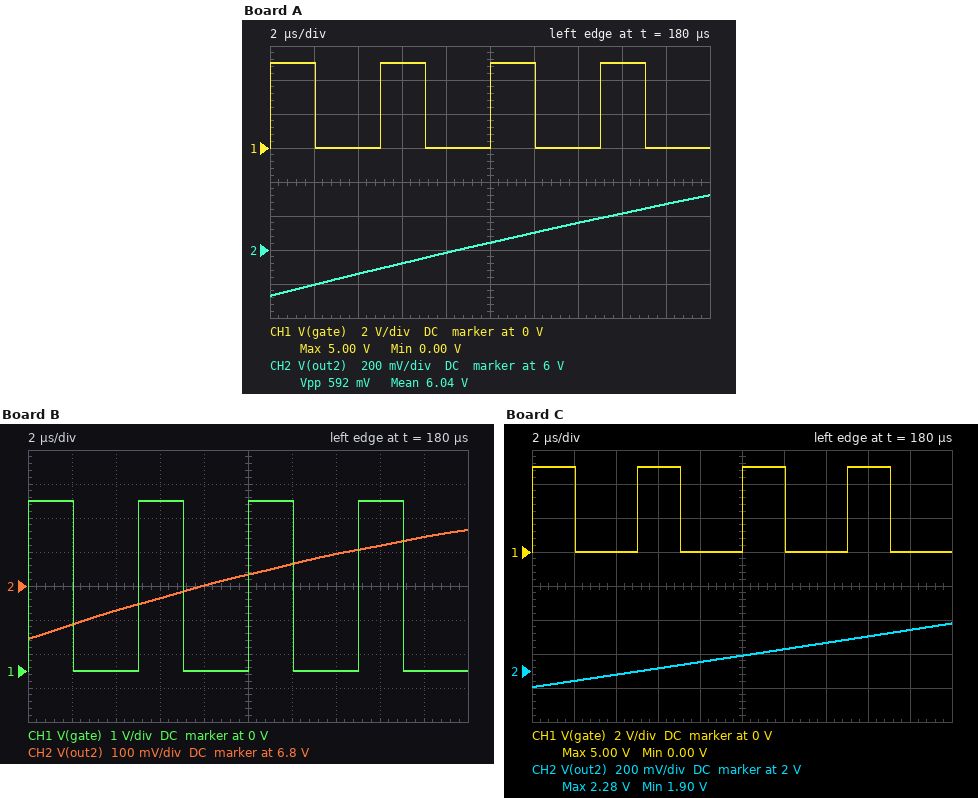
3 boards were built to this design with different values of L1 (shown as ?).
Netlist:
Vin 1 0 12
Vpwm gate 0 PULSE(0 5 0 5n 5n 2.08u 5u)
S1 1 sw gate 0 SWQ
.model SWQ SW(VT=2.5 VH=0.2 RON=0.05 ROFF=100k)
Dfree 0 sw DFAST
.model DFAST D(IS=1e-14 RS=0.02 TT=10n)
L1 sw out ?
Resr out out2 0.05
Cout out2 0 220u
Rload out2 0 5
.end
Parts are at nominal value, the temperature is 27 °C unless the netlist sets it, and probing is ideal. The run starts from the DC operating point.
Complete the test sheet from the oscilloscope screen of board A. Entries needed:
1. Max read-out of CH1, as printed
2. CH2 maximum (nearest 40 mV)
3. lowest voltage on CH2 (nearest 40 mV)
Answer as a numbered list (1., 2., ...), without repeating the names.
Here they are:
1. 5.00 V
2. 6.32 V
3. 5.72 V
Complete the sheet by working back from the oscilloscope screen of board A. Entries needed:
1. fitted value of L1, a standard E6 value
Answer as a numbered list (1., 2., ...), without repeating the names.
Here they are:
1. 33 µH
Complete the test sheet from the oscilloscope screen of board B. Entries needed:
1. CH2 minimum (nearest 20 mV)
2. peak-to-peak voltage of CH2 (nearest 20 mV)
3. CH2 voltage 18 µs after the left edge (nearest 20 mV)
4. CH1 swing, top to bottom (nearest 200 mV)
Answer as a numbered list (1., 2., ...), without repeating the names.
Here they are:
1. 6.64 V
2. 320 mV
3. 6.94 V
4. 5.0 V
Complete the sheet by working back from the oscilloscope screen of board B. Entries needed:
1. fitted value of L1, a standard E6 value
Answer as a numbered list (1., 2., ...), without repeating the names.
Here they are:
1. 22 µH
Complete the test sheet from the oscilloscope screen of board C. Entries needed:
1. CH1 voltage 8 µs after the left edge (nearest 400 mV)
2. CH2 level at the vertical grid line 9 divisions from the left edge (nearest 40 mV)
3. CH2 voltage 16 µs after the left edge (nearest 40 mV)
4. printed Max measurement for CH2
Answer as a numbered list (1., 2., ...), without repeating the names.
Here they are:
1. 0 V
2. 2.24 V
3. 2.20 V
4. 2.28 V
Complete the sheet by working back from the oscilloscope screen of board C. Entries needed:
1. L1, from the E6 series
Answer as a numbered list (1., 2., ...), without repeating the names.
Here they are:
1. 150 µH
